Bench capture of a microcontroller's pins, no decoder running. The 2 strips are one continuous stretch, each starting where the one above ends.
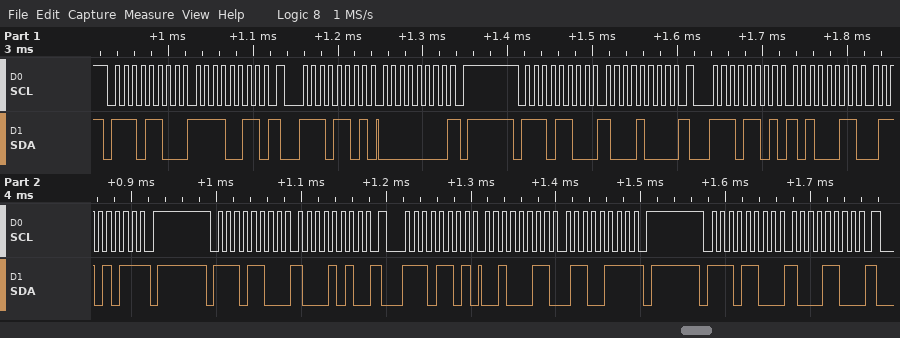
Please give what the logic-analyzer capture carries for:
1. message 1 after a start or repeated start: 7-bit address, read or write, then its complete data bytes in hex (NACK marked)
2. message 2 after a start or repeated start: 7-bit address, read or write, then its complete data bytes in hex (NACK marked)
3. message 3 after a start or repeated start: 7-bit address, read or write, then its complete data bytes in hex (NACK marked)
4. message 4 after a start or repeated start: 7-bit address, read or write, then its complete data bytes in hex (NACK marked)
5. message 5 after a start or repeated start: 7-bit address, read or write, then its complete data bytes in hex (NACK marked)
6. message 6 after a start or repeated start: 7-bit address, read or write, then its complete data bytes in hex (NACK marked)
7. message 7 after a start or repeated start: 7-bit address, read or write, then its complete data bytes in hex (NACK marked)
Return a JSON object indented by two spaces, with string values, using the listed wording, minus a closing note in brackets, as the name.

{
  "message 1 after a start or repeated start: 7-bit address, read or write, then its complete data bytes in hex": "0x76 write: F3",
  "message 2 after a start or repeated start: 7-bit address, read or write, then its complete data bytes in hex": "0x76 read: 00 NACK",
  "message 3 after a start or repeated start: 7-bit address, read or write, then its complete data bytes in hex": "0x76 write: 88",
  "message 4 after a start or repeated start: 7-bit address, read or write, then its complete data bytes in hex": "0x76 read: A3 6B NACK",
  "message 5 after a start or repeated start: 7-bit address, read or write, then its complete data bytes in hex": "0x76 write: 8A",
  "message 6 after a start or repeated start: 7-bit address, read or write, then its complete data bytes in hex": "0x76 read: 23 67 NACK",
  "message 7 after a start or repeated start: 7-bit address, read or write, then its complete data bytes in hex": "0x76 write: 8C"
}
